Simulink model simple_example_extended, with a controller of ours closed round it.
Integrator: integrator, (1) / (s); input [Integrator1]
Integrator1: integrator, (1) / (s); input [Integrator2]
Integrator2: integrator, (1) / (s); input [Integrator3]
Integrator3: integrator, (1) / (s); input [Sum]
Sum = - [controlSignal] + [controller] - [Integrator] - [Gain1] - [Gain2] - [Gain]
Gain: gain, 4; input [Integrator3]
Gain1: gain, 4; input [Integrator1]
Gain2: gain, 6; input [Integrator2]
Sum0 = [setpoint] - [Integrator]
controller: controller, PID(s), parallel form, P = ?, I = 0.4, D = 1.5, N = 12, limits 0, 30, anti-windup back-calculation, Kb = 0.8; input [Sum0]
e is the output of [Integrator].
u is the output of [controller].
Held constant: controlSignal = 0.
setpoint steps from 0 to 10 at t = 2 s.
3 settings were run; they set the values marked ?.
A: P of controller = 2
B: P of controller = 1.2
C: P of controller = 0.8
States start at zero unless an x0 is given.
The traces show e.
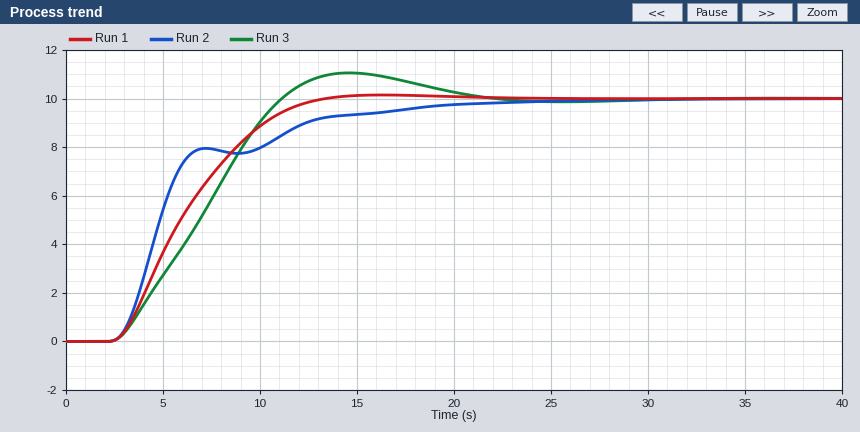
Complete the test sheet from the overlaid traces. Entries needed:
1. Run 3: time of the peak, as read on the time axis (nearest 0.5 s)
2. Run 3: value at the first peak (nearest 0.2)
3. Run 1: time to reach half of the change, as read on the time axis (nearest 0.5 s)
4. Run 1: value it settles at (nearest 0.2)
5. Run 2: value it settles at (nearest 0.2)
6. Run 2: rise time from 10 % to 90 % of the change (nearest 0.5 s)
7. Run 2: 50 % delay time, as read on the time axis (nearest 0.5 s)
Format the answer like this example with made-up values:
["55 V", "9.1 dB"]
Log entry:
["14.5 s", "11.0", "6.0 s", "10.0", "10.0", "9.0 s", "5.0 s"]
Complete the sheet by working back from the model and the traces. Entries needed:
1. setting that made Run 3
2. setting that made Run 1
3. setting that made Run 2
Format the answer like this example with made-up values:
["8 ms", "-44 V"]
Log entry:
["C", "B", "A"]
